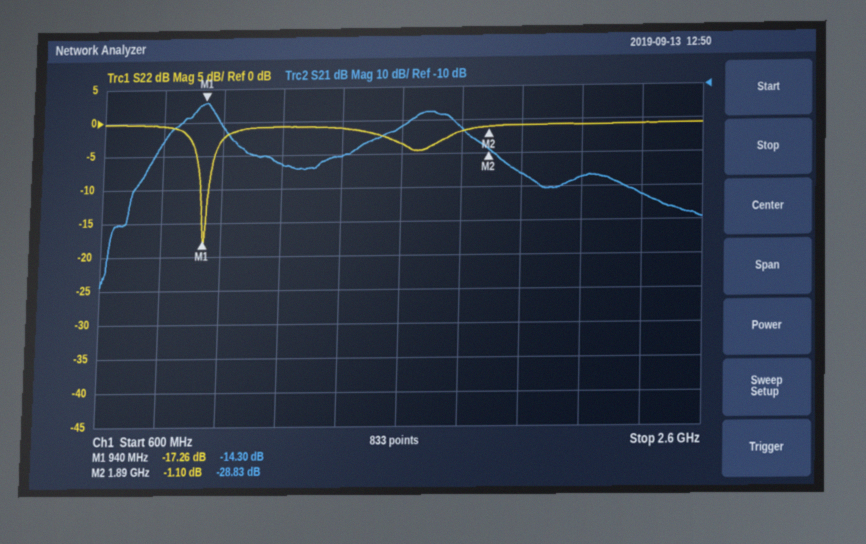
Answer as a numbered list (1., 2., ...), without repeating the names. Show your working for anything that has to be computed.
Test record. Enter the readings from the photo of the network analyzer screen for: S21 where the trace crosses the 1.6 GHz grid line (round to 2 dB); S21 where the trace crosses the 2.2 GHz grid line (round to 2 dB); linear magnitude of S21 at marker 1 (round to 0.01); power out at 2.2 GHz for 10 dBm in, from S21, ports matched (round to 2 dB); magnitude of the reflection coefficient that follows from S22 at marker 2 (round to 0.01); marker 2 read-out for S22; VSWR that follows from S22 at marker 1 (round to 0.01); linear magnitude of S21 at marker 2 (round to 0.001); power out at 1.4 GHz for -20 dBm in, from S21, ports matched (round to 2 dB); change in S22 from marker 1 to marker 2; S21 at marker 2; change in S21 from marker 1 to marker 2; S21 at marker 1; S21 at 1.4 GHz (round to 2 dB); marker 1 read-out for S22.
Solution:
1. -22 dB
2. -38 dB
3. 10^(-14.3/20) ≈ 0.19
4. 10 dBm + (-38 dB) = -28 dBm
5. 10^(-1.1/20) ≈ 0.88
6. -1.10 dB
7. (1 + 0.1371)/(1 − 0.1371) ≈ 1.32
8. 10^(-28.83/20) ≈ 0.036
9. -20 dBm + (-30 dB) = -50 dBm
10. -1.1 − (-17.26) = 16.16 dB
11. -28.83 dB
12. -28.83 − (-14.3) = -14.53 dB
13. -14.30 dB
14. -30 dB
15. -17.26 dB
